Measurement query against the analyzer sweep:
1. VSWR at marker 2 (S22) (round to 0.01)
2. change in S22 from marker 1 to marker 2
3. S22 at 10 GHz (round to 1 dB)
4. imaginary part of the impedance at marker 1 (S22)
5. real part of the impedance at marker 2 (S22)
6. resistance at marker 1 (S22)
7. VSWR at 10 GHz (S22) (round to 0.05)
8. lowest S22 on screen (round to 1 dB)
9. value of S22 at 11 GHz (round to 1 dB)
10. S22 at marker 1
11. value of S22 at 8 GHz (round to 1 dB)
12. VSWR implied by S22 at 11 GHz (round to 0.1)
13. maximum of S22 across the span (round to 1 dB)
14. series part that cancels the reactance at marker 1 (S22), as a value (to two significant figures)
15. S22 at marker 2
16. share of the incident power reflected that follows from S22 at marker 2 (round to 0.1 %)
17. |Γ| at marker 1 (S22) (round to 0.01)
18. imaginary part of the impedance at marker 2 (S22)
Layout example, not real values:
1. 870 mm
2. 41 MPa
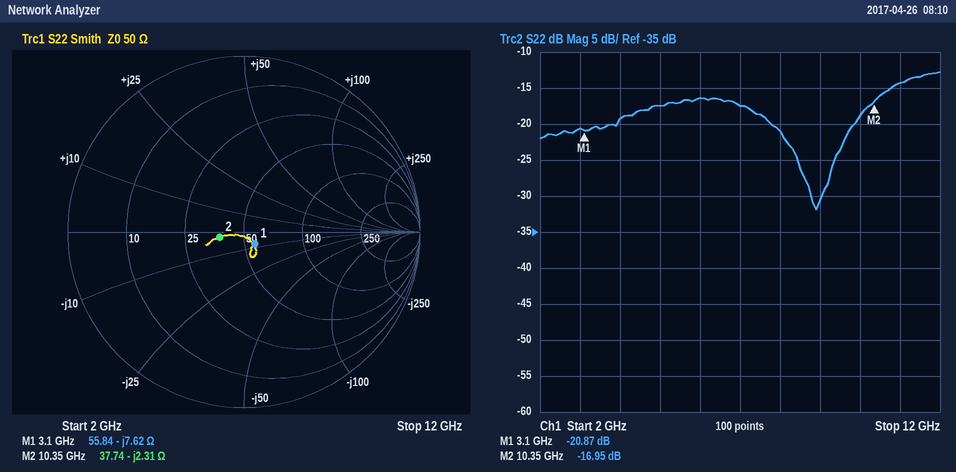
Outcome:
1. 1.33
2. 3.92 dB
3. -19 dB
4. -7.62 Ω
5. 37.74 Ω
6. 55.84 Ω
7. 1.25
8. -32 dB
9. -14 dB
10. -20.87 dB
11. -21 dB
12. 1.5
13. -13 dB
14. 390 pH
15. -16.95 dB
16. 2.0 %
17. 0.09
18. -2.31 Ω
